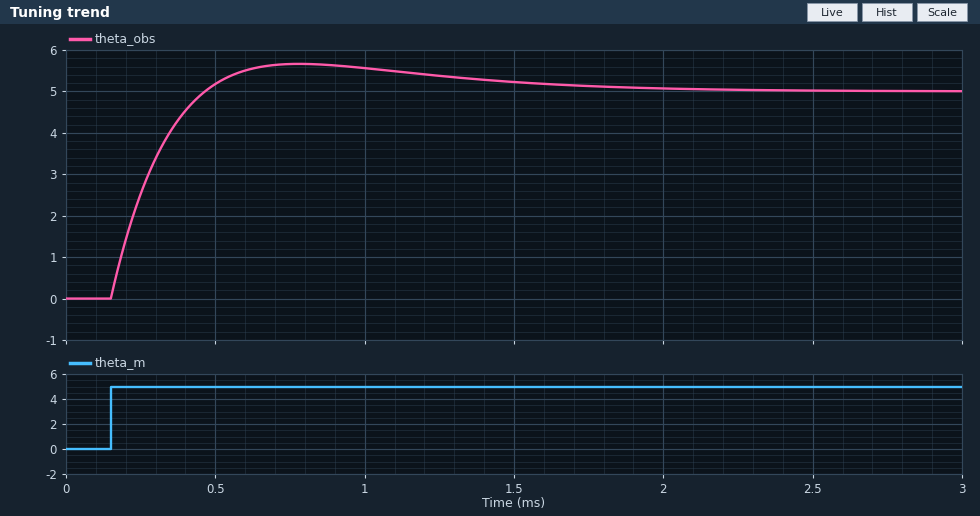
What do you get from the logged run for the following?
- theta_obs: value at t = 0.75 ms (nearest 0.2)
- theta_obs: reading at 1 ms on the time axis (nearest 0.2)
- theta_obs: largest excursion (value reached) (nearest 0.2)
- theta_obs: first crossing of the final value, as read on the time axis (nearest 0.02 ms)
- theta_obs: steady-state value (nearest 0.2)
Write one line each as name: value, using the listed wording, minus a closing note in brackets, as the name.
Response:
theta_obs: value at t = 0.75 ms: 5.6
theta_obs: reading at 1 ms on the time axis: 5.6
theta_obs: largest excursion (value reached): 5.6
theta_obs: first crossing of the final value, as read on the time axis: 0.46 ms
theta_obs: steady-state value: 5.0
